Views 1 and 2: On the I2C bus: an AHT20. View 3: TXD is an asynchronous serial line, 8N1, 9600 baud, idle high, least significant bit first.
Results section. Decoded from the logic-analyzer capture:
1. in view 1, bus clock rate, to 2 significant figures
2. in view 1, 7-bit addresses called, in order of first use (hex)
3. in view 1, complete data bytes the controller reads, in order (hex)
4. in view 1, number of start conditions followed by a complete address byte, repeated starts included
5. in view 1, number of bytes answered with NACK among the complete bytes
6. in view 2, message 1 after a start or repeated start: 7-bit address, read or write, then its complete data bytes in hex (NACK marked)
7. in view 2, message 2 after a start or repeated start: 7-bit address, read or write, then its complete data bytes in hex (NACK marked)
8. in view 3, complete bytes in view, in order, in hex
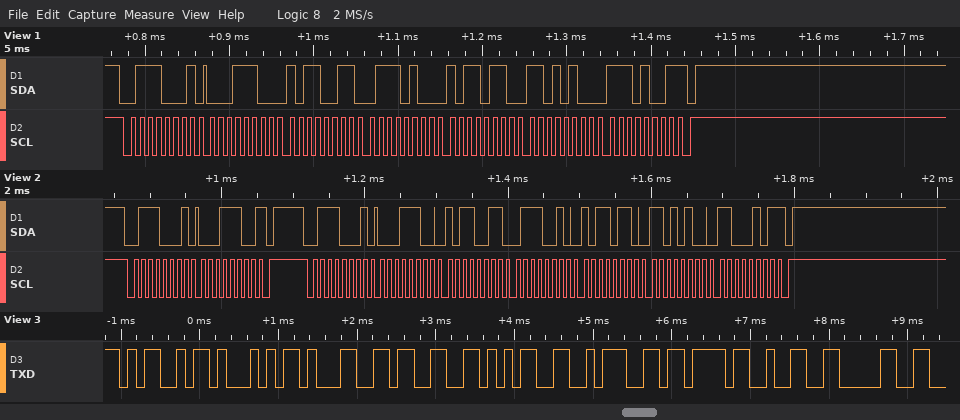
100 kHz
0x38
1C B3 74 B6 D4 E9
1
1
0x38 read: 1C NACK
0x38 read: 1C B3 72 B6 D4 C5 NACK
4D 51 31 33 35 3A 7B 32 30
